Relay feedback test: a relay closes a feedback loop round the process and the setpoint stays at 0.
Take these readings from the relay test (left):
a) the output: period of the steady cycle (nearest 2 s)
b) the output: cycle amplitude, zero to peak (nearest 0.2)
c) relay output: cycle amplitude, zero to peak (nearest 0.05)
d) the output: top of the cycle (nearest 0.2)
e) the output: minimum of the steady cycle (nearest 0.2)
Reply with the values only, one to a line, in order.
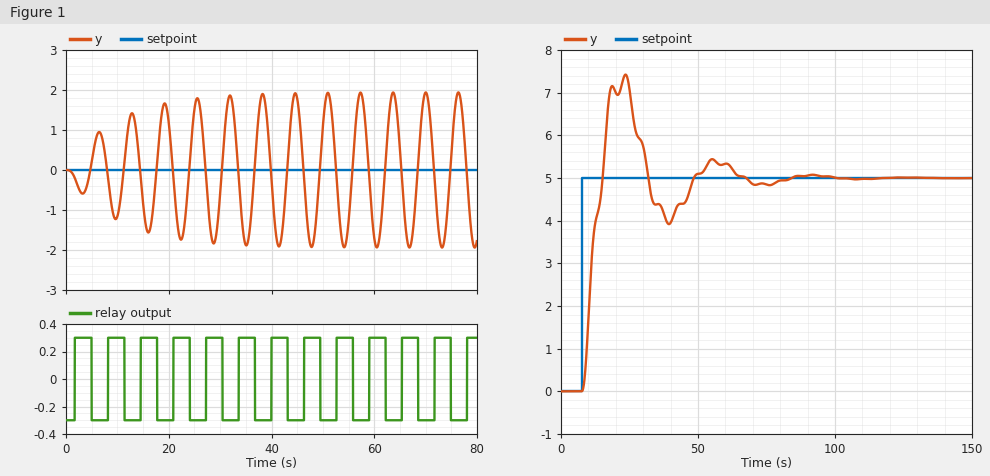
6 s
2.0
0.30
2.0
-2.0
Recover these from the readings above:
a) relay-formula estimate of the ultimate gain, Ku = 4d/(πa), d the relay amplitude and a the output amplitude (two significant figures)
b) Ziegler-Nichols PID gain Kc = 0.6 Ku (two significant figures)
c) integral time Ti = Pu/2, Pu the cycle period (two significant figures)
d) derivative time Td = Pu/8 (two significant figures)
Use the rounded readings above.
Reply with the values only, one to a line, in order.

0.19
0.11
3.0 s
0.75 s
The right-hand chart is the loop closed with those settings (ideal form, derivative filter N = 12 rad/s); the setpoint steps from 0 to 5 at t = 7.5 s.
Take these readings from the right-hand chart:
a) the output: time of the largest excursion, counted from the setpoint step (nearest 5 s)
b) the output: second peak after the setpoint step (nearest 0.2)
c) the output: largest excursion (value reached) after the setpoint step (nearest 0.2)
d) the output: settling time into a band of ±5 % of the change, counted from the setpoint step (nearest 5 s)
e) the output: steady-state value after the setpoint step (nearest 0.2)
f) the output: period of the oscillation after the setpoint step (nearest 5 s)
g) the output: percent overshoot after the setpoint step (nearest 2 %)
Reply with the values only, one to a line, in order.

15 s
5.4
7.4
55 s
5.0
30 s
48 %
